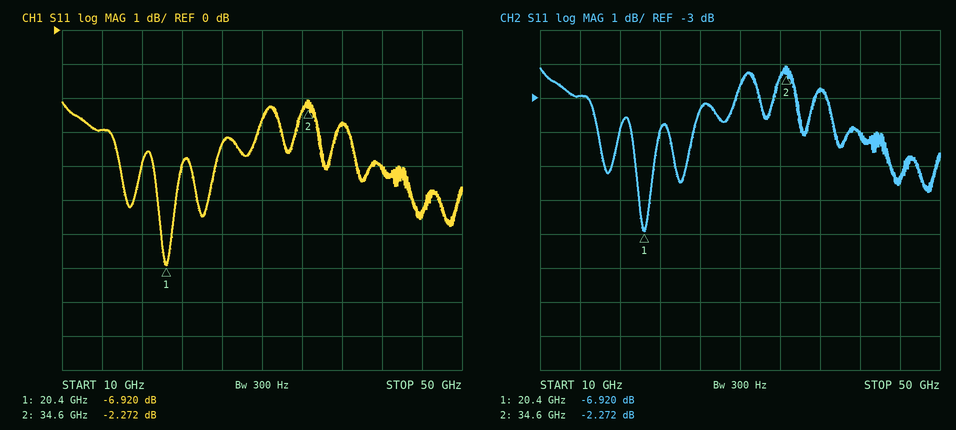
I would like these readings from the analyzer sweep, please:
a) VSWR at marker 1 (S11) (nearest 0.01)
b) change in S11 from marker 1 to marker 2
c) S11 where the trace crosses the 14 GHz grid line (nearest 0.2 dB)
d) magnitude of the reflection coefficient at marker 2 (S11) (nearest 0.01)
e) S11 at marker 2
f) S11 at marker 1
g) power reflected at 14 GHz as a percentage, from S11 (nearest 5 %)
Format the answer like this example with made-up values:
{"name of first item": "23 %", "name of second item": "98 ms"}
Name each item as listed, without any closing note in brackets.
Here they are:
{"VSWR at marker 1 (S11)": "2.64", "change in S11 from marker 1 to marker 2": "4.648 dB", "S11 where the trace crosses the 14 GHz grid line": "-3.0 dB", "magnitude of the reflection coefficient at marker 2 (S11)": "0.77", "S11 at marker 2": "-2.272 dB", "S11 at marker 1": "-6.920 dB", "power reflected at 14 GHz as a percentage, from S11": "50 %"}
